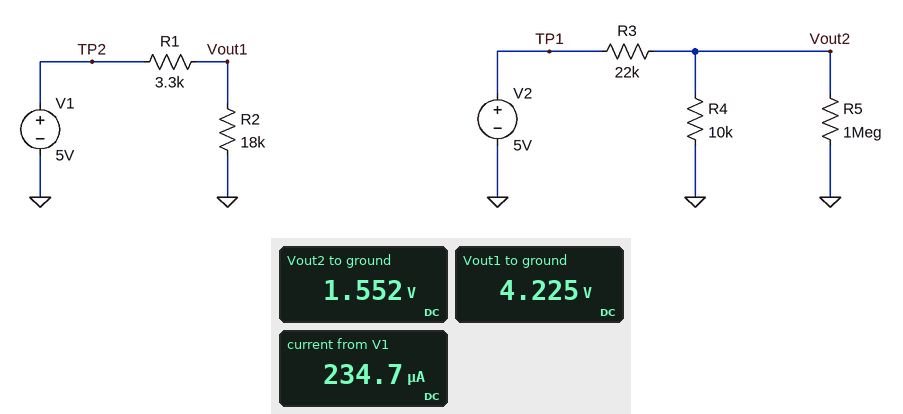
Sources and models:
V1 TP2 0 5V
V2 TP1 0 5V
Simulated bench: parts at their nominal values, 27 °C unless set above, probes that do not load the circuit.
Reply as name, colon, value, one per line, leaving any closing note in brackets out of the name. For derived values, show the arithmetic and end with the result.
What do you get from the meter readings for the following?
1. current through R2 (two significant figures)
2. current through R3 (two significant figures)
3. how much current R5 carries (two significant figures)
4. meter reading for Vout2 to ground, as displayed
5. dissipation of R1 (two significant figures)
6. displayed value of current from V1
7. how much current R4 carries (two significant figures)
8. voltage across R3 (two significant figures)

current through R2: (4.225 V) / 18 kΩ = 230 µA
current through R3: (5 V - 1.552 V) / 22 kΩ = 160 µA
how much current R5 carries: (1.552 V) / 1 MΩ = 1.6 µA
meter reading for Vout2 to ground, as displayed: 1.552 V
dissipation of R1: (5 V - 4.225 V)^2 / 3.3 kΩ = 180 µW
displayed value of current from V1: 234.7 µA
how much current R4 carries: (1.552 V) / 10 kΩ = 160 µA
voltage across R3: 5 V - 1.552 V = 3.4 V
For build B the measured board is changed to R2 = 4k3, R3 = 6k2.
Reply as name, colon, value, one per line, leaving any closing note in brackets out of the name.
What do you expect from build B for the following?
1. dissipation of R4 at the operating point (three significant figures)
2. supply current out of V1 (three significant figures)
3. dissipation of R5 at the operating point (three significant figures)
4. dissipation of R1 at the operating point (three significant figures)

dissipation of R4 at the operating point: 945 µW
supply current out of V1: 658 µA
dissipation of R5 at the operating point: 9.45 µW
dissipation of R1 at the operating point: 1.43 mW
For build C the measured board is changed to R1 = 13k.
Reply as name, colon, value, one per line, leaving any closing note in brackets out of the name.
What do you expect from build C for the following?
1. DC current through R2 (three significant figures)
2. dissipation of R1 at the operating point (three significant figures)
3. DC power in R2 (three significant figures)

DC current through R2: 161 µA
dissipation of R1 at the operating point: 338 µW
DC power in R2: 468 µW
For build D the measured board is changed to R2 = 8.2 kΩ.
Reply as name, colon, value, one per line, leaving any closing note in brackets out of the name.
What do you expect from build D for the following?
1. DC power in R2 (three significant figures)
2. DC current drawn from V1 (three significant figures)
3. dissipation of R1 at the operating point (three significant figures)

DC power in R2: 1.55 mW
DC current drawn from V1: 435 µA
dissipation of R1 at the operating point: 624 µW
